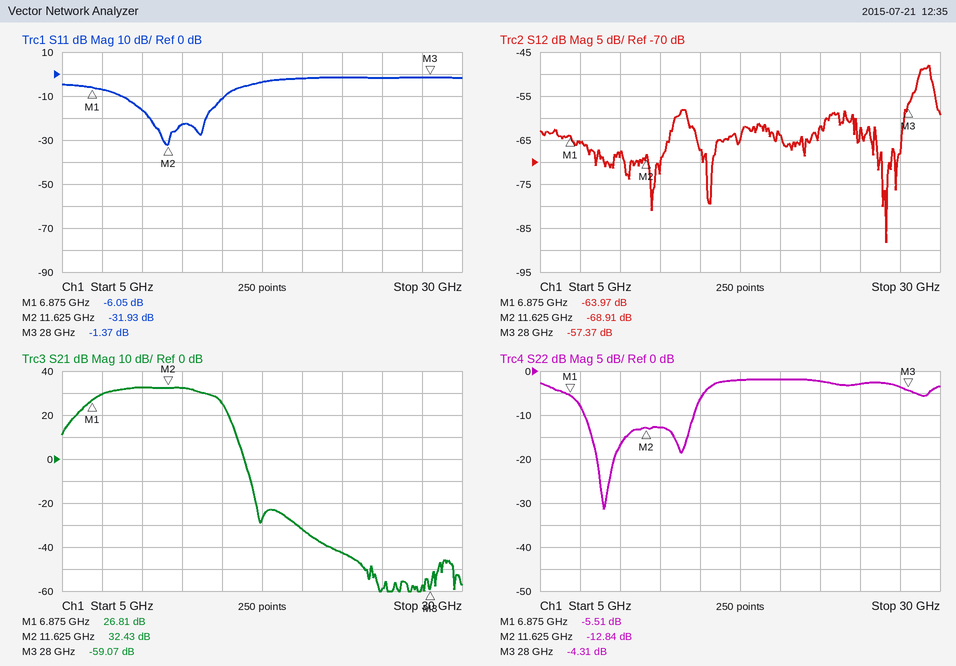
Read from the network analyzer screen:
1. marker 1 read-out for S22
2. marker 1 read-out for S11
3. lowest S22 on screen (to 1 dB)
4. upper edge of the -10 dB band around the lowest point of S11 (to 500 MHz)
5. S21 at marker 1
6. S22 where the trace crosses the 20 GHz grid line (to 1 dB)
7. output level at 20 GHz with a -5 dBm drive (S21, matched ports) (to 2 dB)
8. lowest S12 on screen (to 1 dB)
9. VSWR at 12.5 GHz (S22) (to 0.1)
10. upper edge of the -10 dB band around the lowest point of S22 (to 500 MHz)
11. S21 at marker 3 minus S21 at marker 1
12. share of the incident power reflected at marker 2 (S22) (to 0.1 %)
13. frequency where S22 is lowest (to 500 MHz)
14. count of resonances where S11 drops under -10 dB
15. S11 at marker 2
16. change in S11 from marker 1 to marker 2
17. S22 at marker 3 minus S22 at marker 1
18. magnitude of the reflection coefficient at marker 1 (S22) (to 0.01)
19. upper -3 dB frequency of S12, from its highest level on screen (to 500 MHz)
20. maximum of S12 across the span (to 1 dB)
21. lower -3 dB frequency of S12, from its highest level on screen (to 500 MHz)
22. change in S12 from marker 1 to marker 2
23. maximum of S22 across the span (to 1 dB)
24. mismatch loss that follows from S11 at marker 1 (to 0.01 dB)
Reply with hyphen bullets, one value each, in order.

- -5.51 dB
- -6.05 dB
- -31 dB
- 15.0 GHz
- 26.81 dB
- -2 dB
- -36 dBm
- -88 dB
- 1.6
- 14.5 GHz
- -85.88 dB
- 5.2 %
- 9.0 GHz
- 2
- -31.93 dB
- -25.88 dB
- 1.20 dB
- 0.53
- 29.5 GHz
- -48 dB
- 28.5 GHz
- -4.94 dB
- -2 dB
- 1.24 dB
